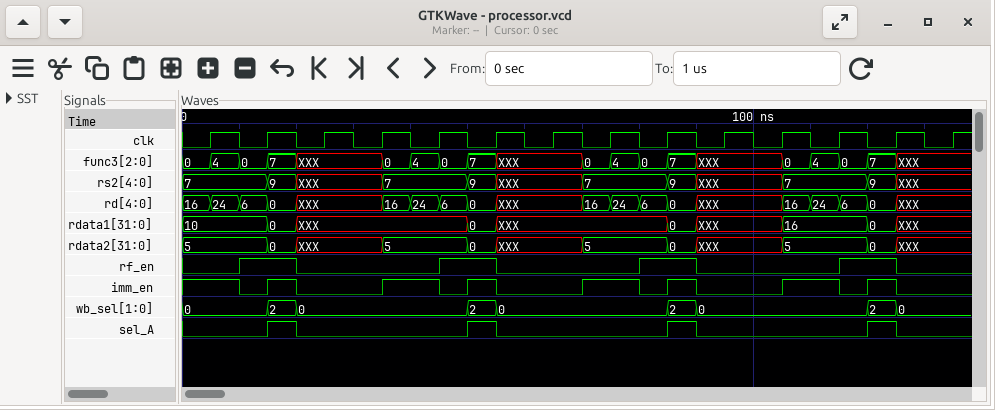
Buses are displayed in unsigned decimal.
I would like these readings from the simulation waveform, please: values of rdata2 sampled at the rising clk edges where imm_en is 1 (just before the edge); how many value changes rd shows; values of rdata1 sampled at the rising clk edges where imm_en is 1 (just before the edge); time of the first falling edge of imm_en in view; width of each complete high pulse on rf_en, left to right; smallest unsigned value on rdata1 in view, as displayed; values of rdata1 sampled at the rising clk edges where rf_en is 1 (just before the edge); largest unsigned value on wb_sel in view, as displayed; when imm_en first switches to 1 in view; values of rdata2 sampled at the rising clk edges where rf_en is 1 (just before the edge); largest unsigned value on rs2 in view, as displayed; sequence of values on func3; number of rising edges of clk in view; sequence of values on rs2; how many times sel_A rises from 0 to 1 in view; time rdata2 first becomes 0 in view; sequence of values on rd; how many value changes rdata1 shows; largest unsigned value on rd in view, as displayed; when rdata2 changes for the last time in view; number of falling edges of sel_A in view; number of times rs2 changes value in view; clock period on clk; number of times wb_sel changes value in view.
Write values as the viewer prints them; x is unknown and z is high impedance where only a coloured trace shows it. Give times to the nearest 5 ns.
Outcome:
5, 5, 0, 5, 5, 0
19
10, XXX, 0, XXX, 16, 0
10 ns
10 ns, 10 ns, 10 ns, 10 ns
0
10, 0, XXX, 0
2
15 ns
5, 0, 5, 0
9
0, 4, 0, 7, XXX, 0, 4, 0, 7, XXX, 0, 4, 0, 7, XXX, 0, 4, 0, 7, XXX
14
7, 9, XXX, 7, 9, XXX, 7, 9, XXX, 7, 9, XXX
4
15 ns
16, 24, 6, 0, XXX, 16, 24, 6, 0, XXX, 16, 24, 6, 0, XXX, 16, 24, 6, 0, XXX
9
24
125 ns
4
11
10 ns
8
